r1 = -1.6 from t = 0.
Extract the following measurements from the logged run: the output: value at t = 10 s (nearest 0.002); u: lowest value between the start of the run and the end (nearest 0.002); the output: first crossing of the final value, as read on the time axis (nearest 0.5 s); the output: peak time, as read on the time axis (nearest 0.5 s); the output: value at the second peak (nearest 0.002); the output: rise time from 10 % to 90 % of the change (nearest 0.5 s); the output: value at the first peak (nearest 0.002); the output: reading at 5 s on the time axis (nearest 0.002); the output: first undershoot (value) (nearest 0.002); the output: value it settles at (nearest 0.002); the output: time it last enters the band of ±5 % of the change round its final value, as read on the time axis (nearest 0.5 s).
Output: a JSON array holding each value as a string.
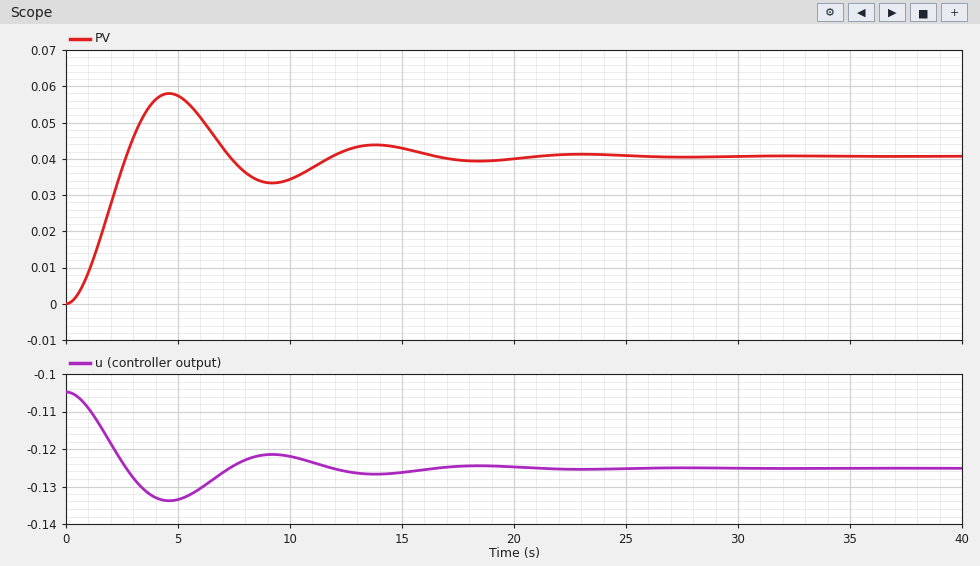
["0.034", "-0.134", "2.5 s", "4.5 s", "0.044", "2.0 s", "0.058", "0.058", "0.034", "0.040", "15.0 s"]
